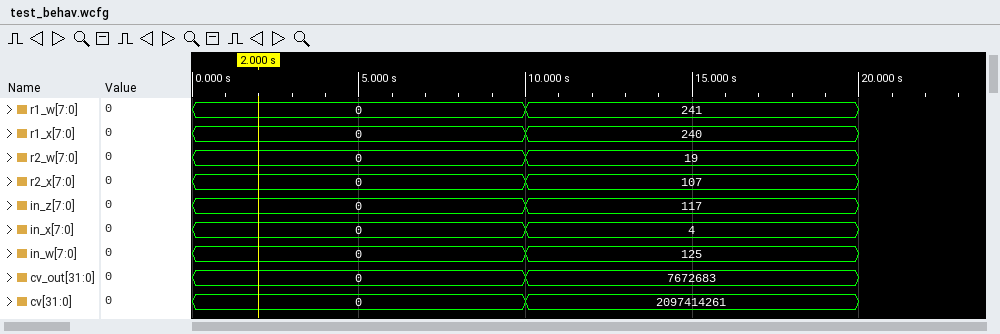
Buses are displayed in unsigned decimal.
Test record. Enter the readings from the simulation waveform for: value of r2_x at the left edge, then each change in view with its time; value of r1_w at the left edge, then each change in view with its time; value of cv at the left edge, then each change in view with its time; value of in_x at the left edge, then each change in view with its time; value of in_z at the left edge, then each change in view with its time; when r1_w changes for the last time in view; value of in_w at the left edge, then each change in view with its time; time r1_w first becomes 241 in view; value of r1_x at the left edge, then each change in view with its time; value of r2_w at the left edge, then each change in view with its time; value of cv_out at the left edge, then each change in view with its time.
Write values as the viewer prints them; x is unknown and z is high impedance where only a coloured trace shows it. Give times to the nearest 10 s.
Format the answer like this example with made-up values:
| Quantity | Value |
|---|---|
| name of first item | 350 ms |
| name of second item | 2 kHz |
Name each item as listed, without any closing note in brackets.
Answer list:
| Quantity | Value |
|---|---|
| value of r2_x at the left edge, then each change in view with its time | 0, 107 at 10 s |
| value of r1_w at the left edge, then each change in view with its time | 0, 241 at 10 s |
| value of cv at the left edge, then each change in view with its time | 0, 2097414261 at 10 s |
| value of in_x at the left edge, then each change in view with its time | 0, 4 at 10 s |
| value of in_z at the left edge, then each change in view with its time | 0, 117 at 10 s |
| when r1_w changes for the last time in view | 10 s |
| value of in_w at the left edge, then each change in view with its time | 0, 125 at 10 s |
| time r1_w first becomes 241 in view | 10 s |
| value of r1_x at the left edge, then each change in view with its time | 0, 240 at 10 s |
| value of r2_w at the left edge, then each change in view with its time | 0, 19 at 10 s |
| value of cv_out at the left edge, then each change in view with its time | 0, 7672683 at 10 s |
